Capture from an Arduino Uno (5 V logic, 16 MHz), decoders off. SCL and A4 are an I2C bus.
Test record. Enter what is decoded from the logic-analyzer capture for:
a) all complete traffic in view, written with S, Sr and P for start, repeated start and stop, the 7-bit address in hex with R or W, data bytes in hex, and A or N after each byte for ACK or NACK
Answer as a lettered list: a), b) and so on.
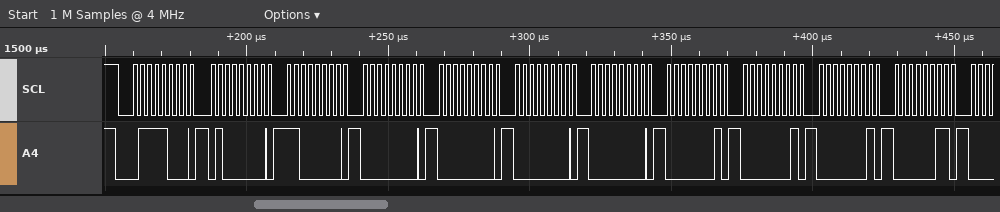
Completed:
a) S 3CW A 40 A C0 A 00 A 00 A 00 A 00 A 01 A 01 A 01 A 03 A
